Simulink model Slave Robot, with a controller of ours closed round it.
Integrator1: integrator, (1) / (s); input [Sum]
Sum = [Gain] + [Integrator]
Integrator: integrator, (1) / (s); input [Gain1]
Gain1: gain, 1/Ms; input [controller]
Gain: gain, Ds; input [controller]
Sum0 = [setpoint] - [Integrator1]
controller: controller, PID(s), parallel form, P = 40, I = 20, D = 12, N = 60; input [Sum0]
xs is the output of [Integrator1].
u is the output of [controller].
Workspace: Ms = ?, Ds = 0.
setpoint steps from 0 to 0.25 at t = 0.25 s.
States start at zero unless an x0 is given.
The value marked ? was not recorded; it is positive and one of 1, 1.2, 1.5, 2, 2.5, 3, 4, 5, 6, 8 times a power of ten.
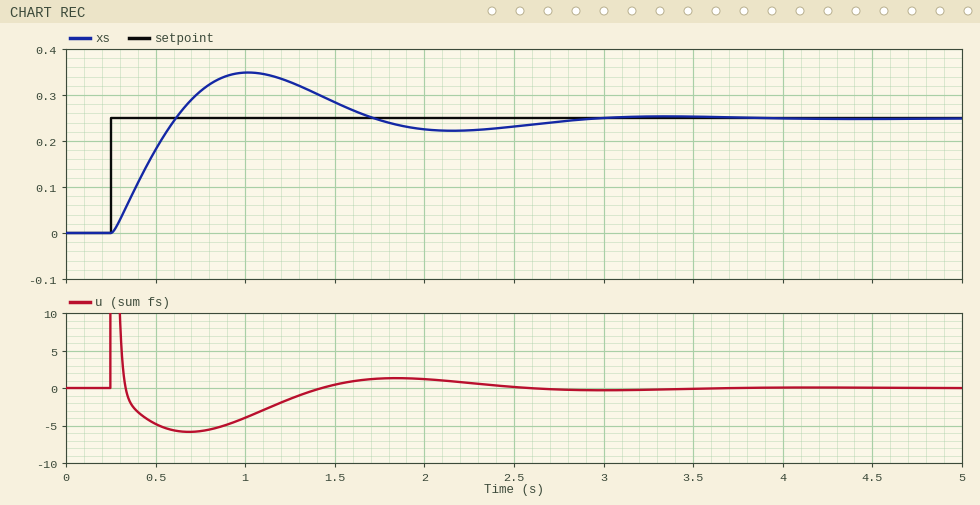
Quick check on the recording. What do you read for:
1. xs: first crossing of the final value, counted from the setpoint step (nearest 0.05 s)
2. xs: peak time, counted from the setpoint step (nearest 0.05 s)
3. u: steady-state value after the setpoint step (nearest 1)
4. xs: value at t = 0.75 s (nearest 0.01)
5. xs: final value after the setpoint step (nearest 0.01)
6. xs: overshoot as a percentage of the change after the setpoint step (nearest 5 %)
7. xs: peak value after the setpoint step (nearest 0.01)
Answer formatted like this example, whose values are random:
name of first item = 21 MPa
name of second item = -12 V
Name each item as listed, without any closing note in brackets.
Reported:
xs: first crossing of the final value, counted from the setpoint step = 0.35 s
xs: peak time, counted from the setpoint step = 0.75 s
u: steady-state value after the setpoint step = 0
xs: value at t = 0.75 s = 0.31
xs: final value after the setpoint step = 0.25
xs: overshoot as a percentage of the change after the setpoint step = 40 %
xs: peak value after the setpoint step = 0.35
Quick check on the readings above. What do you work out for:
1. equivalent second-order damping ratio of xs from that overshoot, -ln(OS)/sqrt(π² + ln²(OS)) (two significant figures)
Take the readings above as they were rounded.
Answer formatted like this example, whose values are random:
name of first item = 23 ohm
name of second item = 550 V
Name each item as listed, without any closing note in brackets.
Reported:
equivalent second-order damping ratio of xs from that overshoot, -ln(OS)/sqrt(π² + ln²(OS)) = 0.28
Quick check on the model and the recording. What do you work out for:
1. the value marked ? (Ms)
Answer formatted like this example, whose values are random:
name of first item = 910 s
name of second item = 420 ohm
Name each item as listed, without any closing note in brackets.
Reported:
the value marked ? = 4
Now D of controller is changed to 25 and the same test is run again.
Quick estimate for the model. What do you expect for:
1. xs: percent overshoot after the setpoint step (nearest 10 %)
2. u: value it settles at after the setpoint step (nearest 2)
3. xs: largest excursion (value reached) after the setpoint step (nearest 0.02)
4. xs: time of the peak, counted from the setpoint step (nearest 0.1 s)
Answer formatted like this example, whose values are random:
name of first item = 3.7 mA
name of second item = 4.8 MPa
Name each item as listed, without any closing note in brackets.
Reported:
xs: percent overshoot after the setpoint step = 20 %
u: value it settles at after the setpoint step = 0
xs: largest excursion (value reached) after the setpoint step = 0.30
xs: time of the peak, counted from the setpoint step = 0.6 s
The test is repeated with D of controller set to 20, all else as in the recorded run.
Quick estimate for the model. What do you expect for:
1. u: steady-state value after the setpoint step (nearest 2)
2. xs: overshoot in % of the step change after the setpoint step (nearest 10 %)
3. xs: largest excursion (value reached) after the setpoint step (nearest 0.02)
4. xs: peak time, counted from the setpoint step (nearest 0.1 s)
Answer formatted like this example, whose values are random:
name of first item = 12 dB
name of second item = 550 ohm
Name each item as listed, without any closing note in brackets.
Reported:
u: steady-state value after the setpoint step = 0
xs: overshoot in % of the step change after the setpoint step = 20 %
xs: largest excursion (value reached) after the setpoint step = 0.30
xs: peak time, counted from the setpoint step = 0.7 s
